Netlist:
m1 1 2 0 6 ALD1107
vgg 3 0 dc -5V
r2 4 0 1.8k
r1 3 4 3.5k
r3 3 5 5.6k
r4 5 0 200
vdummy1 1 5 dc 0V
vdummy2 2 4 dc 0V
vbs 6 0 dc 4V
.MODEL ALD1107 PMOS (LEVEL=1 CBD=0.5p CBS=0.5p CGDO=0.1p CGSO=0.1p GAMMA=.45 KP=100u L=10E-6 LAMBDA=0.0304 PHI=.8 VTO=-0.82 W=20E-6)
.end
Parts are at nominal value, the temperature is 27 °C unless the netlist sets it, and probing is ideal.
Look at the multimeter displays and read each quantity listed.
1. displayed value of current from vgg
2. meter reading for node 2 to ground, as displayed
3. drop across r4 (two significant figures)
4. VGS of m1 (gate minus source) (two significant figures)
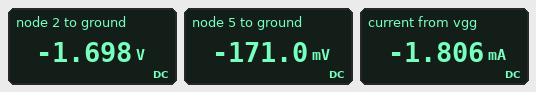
-1.806 mA
-1.698 V
170 mV
-1.7 V
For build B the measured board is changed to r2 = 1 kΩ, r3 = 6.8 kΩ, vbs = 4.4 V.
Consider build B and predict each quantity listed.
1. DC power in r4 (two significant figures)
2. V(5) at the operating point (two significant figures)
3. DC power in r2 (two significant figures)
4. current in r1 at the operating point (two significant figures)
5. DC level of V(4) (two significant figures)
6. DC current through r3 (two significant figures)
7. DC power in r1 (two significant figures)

100 µW
-140 mV
1.2 mW
1.1 mA
-1.1 V
710 µA
4.3 mW
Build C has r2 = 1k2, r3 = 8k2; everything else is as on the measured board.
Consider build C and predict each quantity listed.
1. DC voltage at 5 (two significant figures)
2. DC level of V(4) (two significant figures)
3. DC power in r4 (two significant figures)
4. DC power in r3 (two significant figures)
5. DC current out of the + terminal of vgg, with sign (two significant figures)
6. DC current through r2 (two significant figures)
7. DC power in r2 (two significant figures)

-120 mV
-1.3 V
71 µW
2.9 mW
-1.7 mA
1.1 mA
1.4 mW
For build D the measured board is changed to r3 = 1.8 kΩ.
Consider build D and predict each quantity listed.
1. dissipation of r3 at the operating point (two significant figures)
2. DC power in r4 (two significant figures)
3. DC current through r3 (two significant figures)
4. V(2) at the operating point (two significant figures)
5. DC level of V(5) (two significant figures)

11 mW
1.2 mW
2.5 mA
-1.7 V
-500 mV
